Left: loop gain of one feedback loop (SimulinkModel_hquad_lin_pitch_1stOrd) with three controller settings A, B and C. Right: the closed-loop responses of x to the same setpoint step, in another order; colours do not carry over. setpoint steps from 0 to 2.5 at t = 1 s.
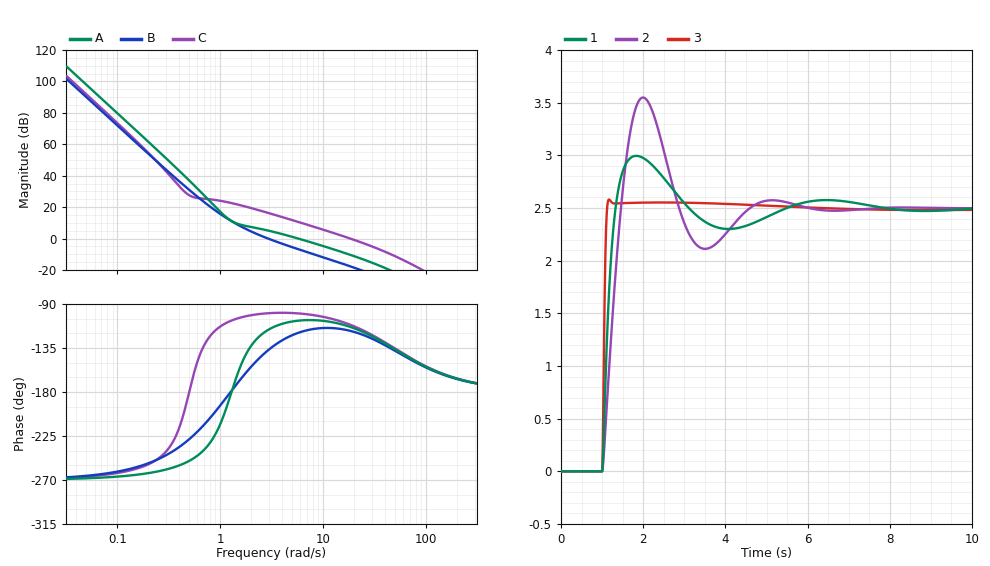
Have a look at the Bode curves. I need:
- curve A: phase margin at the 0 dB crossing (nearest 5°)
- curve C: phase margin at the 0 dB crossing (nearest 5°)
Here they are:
75°
70°
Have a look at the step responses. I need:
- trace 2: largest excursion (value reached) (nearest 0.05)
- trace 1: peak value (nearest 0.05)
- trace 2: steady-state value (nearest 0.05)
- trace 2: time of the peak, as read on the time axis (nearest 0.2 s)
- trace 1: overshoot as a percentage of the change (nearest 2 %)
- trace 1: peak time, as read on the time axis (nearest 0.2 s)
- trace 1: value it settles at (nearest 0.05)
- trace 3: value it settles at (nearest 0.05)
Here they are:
3.55
3.00
2.50
2.0 s
20 %
1.8 s
2.50
2.50
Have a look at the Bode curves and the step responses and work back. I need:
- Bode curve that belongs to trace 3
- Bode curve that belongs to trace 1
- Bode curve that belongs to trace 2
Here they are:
C
A
B
